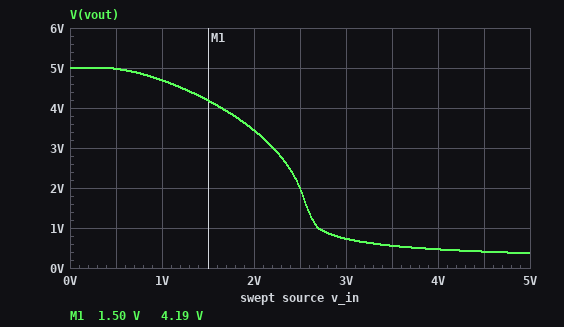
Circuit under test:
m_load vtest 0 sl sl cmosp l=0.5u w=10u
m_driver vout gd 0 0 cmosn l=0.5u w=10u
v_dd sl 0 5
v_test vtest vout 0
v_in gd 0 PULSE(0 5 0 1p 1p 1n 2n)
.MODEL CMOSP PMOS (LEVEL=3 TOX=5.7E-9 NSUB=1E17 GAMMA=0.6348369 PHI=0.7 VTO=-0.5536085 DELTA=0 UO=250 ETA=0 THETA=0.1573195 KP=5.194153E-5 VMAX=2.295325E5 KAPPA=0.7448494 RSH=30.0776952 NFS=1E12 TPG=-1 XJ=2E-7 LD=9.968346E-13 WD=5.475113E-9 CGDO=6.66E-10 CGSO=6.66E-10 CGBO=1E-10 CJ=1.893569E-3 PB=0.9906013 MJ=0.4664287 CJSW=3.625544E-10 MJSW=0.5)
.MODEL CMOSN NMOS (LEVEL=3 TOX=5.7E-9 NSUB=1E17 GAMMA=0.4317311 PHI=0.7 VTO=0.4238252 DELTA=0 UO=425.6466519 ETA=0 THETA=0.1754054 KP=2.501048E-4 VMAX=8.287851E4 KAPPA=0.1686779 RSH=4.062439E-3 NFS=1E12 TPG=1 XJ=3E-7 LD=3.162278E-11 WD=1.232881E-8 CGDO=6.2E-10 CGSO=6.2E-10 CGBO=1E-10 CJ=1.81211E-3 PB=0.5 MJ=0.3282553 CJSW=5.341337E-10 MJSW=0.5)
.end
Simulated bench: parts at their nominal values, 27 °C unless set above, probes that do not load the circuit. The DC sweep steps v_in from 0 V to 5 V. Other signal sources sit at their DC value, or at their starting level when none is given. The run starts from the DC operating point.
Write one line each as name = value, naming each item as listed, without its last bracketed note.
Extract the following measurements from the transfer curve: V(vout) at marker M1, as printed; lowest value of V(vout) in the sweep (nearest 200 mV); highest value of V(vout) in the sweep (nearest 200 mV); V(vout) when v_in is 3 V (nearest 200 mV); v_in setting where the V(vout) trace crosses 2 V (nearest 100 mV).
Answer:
V(vout) at marker M1, as printed = 4.19 V
lowest value of V(vout) in the sweep = 400 mV
highest value of V(vout) in the sweep = 5.0 V
V(vout) when v_in is 3 V = 800 mV
v_in setting where the V(vout) trace crosses 2 V = 2.5 V
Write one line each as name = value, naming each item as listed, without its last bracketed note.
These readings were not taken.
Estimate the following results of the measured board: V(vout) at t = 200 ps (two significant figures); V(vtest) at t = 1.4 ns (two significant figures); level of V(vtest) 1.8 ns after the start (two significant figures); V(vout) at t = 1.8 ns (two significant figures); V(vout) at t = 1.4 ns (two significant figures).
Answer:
V(vout) at t = 200 ps = 370 mV
V(vtest) at t = 1.4 ns = 5.0 V
level of V(vtest) 1.8 ns after the start = 5.0 V
V(vout) at t = 1.8 ns = 5.0 V
V(vout) at t = 1.4 ns = 5.0 V
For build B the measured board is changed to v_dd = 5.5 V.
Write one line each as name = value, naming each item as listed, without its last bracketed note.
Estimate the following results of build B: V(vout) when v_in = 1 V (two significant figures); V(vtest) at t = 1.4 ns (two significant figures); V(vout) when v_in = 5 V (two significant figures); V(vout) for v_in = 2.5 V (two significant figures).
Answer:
V(vout) when v_in = 1 V = 5.2 V
V(vtest) at t = 1.4 ns = 5.5 V
V(vout) when v_in = 5 V = 450 mV
V(vout) for v_in = 2.5 V = 3.1 V
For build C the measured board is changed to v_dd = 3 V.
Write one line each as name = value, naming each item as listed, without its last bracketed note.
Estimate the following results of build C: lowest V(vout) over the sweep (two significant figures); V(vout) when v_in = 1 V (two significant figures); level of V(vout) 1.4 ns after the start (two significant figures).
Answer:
lowest V(vout) over the sweep = 130 mV
V(vout) when v_in = 1 V = 2.6 V
level of V(vout) 1.4 ns after the start = 3.0 V
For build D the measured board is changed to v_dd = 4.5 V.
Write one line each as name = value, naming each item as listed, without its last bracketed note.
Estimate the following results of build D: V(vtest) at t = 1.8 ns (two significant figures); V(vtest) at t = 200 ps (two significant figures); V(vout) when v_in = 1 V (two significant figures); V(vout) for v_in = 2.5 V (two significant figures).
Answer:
V(vtest) at t = 1.8 ns = 4.5 V
V(vtest) at t = 200 ps = 300 mV
V(vout) when v_in = 1 V = 4.2 V
V(vout) for v_in = 2.5 V = 810 mV
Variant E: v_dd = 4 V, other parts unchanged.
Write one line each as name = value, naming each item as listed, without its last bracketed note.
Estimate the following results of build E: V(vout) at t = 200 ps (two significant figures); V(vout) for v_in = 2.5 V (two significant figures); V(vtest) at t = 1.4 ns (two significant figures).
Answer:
V(vout) at t = 200 ps = 240 mV
V(vout) for v_in = 2.5 V = 540 mV
V(vtest) at t = 1.4 ns = 4.0 V
